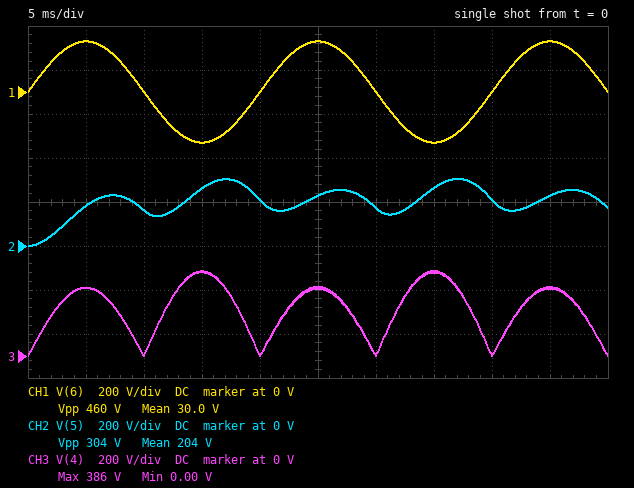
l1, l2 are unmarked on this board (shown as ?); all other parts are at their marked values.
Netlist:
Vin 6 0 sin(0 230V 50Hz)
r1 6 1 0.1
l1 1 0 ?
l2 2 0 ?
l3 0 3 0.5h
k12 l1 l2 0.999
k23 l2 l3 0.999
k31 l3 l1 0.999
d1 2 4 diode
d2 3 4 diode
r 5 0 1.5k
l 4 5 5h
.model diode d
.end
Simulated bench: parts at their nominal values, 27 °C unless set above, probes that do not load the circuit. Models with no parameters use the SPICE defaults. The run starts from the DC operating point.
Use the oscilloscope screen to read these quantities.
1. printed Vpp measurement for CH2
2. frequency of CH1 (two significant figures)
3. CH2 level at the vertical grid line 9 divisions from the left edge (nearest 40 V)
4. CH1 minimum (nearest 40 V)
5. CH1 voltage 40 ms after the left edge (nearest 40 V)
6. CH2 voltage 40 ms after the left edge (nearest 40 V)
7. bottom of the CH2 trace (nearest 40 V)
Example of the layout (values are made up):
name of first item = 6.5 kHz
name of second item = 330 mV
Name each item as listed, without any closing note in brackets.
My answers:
printed Vpp measurement for CH2 = 304 V
frequency of CH1 = 50 Hz
CH2 level at the vertical grid line 9 divisions from the left edge = 240 V
CH1 minimum = -240 V
CH1 voltage 40 ms after the left edge = 0 V
CH2 voltage 40 ms after the left edge = 200 V
bottom of the CH2 trace = 0 V
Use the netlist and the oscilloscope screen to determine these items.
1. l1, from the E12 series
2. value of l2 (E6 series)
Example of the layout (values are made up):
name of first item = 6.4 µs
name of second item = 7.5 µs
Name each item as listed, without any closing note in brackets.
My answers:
l1, from the E12 series = 180 mH
value of l2 = 330 mH
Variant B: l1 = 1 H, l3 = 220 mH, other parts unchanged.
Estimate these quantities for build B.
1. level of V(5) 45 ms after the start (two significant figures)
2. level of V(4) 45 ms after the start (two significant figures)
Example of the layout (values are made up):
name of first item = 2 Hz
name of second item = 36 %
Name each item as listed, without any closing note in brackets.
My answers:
level of V(5) 45 ms after the start = 90 V
level of V(4) 45 ms after the start = 130 V
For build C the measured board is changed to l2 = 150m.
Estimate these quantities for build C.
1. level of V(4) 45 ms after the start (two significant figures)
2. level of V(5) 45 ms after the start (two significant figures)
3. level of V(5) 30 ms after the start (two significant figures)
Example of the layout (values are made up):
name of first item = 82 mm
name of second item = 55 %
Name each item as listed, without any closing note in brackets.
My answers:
level of V(4) 45 ms after the start = 210 V
level of V(5) 45 ms after the start = 170 V
level of V(5) 30 ms after the start = 120 V
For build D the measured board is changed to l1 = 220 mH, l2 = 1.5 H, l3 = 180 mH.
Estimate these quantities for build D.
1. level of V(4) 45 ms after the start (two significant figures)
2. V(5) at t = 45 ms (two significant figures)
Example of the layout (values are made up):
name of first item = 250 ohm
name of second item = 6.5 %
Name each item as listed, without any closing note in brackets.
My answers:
level of V(4) 45 ms after the start = 600 V
V(5) at t = 45 ms = 380 V
